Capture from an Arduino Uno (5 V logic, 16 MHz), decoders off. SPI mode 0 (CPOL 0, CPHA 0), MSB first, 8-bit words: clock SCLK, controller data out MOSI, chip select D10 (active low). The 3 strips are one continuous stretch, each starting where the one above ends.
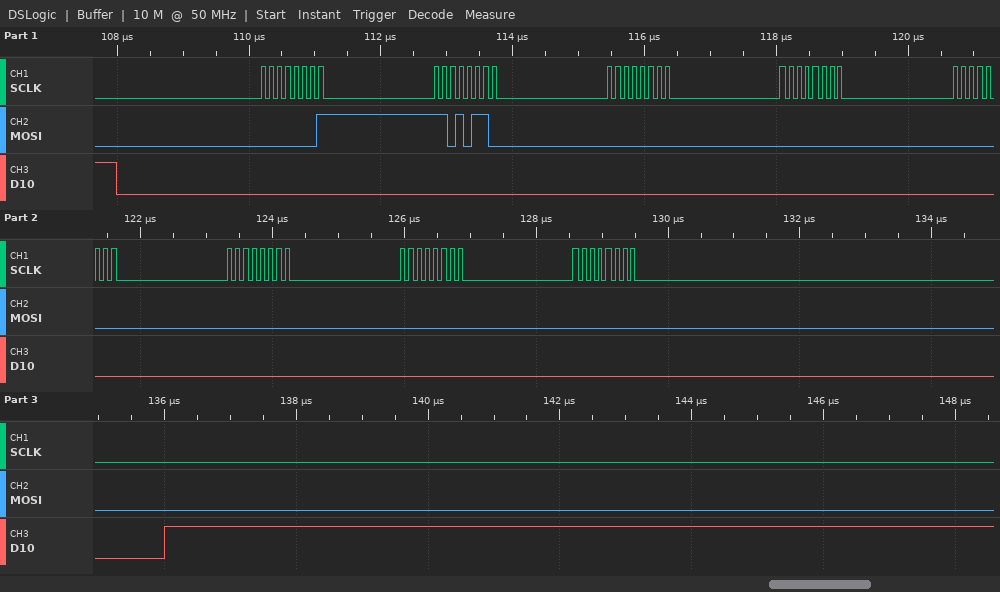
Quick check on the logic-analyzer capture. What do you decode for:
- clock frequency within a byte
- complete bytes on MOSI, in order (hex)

8 MHz
01 D6 00 00 00 00 00 00
